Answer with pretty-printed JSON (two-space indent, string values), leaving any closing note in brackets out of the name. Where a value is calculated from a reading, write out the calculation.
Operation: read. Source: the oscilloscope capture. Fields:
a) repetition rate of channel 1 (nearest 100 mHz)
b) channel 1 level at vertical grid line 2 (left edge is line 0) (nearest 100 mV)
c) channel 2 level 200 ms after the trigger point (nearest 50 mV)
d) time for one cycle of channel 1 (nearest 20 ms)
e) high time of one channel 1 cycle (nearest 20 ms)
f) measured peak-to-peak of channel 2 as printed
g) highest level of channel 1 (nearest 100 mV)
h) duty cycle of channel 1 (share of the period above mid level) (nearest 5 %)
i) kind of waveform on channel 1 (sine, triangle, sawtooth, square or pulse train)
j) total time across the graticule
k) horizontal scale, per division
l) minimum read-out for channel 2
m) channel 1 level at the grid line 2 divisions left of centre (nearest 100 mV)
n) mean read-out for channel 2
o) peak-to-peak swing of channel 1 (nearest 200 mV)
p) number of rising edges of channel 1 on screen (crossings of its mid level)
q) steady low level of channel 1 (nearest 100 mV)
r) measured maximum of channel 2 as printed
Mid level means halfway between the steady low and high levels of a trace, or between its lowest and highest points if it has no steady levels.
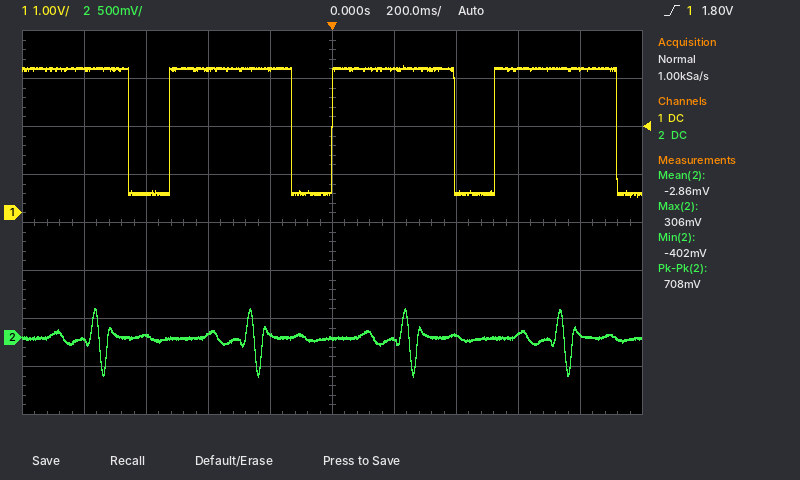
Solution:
{
  "repetition rate of channel 1": "1 / 520 ms ≈ 1.9 Hz",
  "channel 1 level at vertical grid line 2 (left edge is line 0)": "400 mV",
  "channel 2 level 200 ms after the trigger point": "-50 mV",
  "time for one cycle of channel 1": "520 ms",
  "high time of one channel 1 cycle": "400 ms",
  "measured peak-to-peak of channel 2 as printed": "708 mV",
  "highest level of channel 1": "3.1 V",
  "duty cycle of channel 1 (share of the period above mid level)": "400 ms / 520 ms ≈ 76.9 %, so 75 % to the nearest 5 %",
  "kind of waveform on channel 1": "pulse train",
  "total time across the graticule": "2 s",
  "horizontal scale, per division": "200 ms",
  "minimum read-out for channel 2": "-402 mV",
  "channel 1 level at the grid line 2 divisions left of centre": "3.0 V",
  "mean read-out for channel 2": "-2.86 mV",
  "peak-to-peak swing of channel 1": "2.8 V",
  "number of rising edges of channel 1 on screen": "3",
  "steady low level of channel 1": "400 mV",
  "measured maximum of channel 2 as printed": "306 mV"
}
